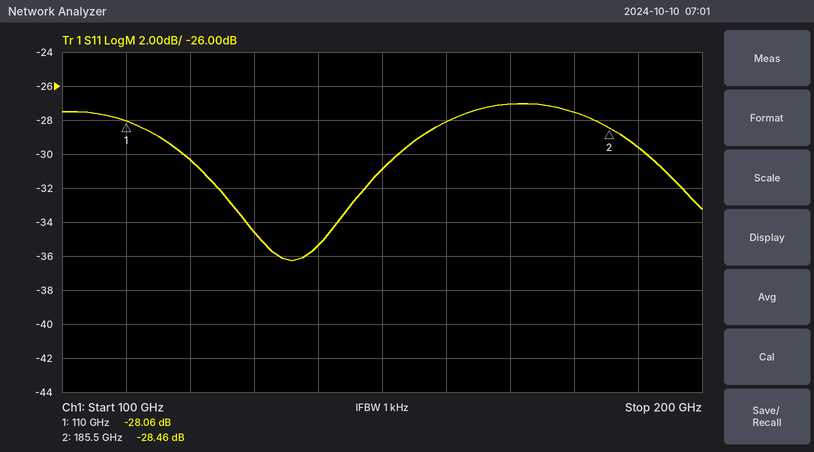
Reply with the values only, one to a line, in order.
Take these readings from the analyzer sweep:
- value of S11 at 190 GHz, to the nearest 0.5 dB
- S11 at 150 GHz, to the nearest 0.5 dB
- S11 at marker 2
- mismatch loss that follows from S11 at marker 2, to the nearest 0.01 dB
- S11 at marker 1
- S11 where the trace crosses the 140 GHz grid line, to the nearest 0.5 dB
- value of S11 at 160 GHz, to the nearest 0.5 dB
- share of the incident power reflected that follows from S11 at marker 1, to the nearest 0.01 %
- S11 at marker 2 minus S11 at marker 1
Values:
-29.5 dB
-31.0 dB
-28.46 dB
0.01 dB
-28.06 dB
-35.5 dB
-28.0 dB
0.16 %
-0.40 dB
